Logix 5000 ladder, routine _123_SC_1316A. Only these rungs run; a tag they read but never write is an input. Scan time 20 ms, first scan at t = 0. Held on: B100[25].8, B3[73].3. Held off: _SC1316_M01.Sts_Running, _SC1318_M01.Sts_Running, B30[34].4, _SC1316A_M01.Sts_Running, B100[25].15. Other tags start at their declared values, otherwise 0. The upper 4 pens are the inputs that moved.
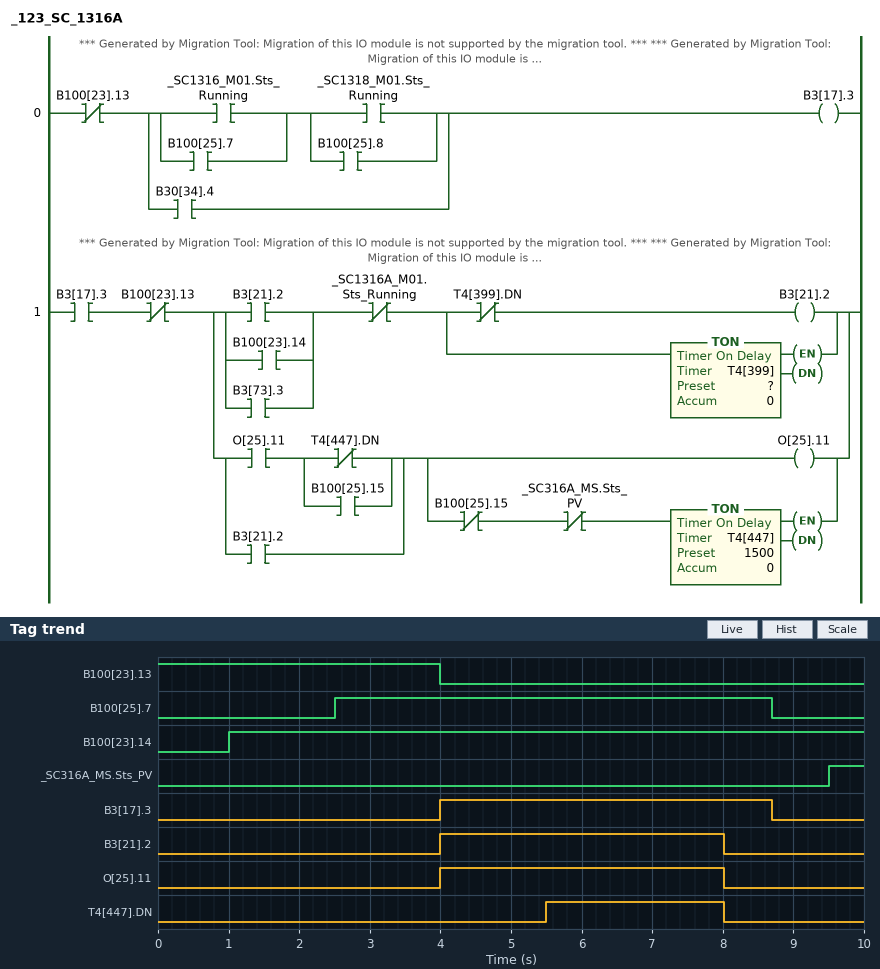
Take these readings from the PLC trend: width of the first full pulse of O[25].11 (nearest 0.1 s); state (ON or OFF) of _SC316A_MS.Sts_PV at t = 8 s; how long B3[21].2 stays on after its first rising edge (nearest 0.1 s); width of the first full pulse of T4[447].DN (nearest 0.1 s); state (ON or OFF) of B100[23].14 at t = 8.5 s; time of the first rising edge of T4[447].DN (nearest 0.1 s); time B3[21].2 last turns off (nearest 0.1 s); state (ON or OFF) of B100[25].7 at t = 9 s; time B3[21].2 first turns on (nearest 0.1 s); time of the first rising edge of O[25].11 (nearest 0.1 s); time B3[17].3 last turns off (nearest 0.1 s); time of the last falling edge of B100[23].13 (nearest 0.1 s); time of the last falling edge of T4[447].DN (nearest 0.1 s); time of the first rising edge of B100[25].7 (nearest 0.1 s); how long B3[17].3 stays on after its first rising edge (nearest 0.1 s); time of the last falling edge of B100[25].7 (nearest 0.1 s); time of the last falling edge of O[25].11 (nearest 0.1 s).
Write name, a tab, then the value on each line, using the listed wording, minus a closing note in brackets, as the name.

width of the first full pulse of O[25].11	4.0 s
state (ON or OFF) of _SC316A_MS.Sts_PV at t = 8 s	OFF
how long B3[21].2 stays on after its first rising edge	4.0 s
width of the first full pulse of T4[447].DN	2.5 s
state (ON or OFF) of B100[23].14 at t = 8.5 s	ON
time of the first rising edge of T4[447].DN	5.5 s
time B3[21].2 last turns off	8.0 s
state (ON or OFF) of B100[25].7 at t = 9 s	OFF
time B3[21].2 first turns on	4.0 s
time of the first rising edge of O[25].11	4.0 s
time B3[17].3 last turns off	8.7 s
time of the last falling edge of B100[23].13	4.0 s
time of the last falling edge of T4[447].DN	8.0 s
time of the first rising edge of B100[25].7	2.5 s
how long B3[17].3 stays on after its first rising edge	4.7 s
time of the last falling edge of B100[25].7	8.7 s
time of the last falling edge of O[25].11	8.0 s
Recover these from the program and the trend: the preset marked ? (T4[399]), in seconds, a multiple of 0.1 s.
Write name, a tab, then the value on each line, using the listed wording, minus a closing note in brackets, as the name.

the preset marked ? (T4[399]), in seconds, a multiple of 0.1 s	4.0 s
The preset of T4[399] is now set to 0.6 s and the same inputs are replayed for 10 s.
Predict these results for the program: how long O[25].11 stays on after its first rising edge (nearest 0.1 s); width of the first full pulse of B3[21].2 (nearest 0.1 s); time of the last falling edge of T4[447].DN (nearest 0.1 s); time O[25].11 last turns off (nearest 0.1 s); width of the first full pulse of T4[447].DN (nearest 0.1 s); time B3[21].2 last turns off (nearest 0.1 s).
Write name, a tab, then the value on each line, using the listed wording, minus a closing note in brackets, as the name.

how long O[25].11 stays on after its first rising edge	1.5 s
width of the first full pulse of B3[21].2	0.6 s
time of the last falling edge of T4[447].DN	5.5 s
time O[25].11 last turns off	5.5 s
width of the first full pulse of T4[447].DN	0.0 s
time B3[21].2 last turns off	4.6 s
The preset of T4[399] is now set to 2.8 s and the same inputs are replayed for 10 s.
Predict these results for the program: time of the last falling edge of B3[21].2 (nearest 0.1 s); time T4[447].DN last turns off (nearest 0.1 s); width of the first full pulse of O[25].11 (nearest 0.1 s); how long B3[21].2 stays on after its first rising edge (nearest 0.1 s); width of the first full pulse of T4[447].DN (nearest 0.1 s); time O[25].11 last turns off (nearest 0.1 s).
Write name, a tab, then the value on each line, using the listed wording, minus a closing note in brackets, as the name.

time of the last falling edge of B3[21].2	6.8 s
time T4[447].DN last turns off	6.8 s
width of the first full pulse of O[25].11	2.8 s
how long B3[21].2 stays on after its first rising edge	2.8 s
width of the first full pulse of T4[447].DN	1.3 s
time O[25].11 last turns off	6.8 s
